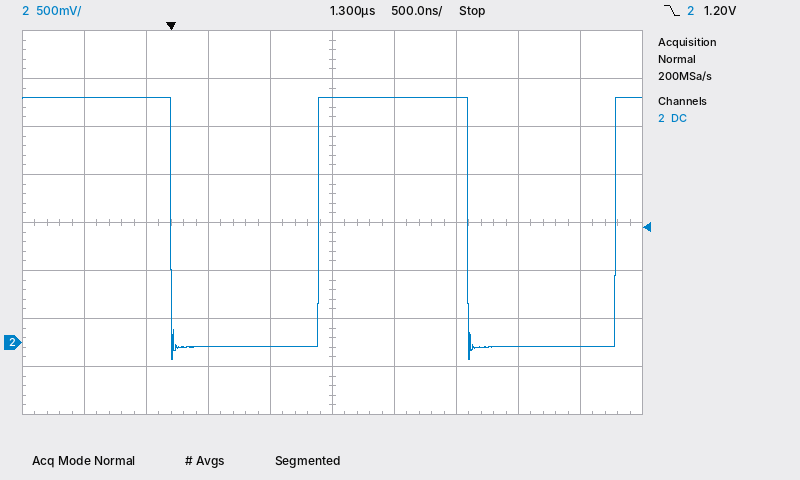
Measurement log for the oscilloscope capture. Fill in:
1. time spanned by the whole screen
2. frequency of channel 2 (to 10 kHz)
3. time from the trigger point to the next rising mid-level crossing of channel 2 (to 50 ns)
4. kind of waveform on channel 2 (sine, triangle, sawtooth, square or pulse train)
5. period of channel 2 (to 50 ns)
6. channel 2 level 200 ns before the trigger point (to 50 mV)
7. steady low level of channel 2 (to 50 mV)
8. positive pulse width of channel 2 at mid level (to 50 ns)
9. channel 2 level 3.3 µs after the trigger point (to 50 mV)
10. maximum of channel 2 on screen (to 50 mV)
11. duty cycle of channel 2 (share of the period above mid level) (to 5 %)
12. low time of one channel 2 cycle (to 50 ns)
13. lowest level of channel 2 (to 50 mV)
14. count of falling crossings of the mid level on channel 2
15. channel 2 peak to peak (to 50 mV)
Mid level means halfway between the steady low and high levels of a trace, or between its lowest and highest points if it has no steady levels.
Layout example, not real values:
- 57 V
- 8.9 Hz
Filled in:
- 5 µs
- 420 kHz
- 1.20 µs
- square
- 2.40 µs
- 2.55 V
- -50 mV
- 1.20 µs
- -50 mV
- 2.55 V
- 50 %
- 1.20 µs
- -200 mV
- 2
- 2.75 V
